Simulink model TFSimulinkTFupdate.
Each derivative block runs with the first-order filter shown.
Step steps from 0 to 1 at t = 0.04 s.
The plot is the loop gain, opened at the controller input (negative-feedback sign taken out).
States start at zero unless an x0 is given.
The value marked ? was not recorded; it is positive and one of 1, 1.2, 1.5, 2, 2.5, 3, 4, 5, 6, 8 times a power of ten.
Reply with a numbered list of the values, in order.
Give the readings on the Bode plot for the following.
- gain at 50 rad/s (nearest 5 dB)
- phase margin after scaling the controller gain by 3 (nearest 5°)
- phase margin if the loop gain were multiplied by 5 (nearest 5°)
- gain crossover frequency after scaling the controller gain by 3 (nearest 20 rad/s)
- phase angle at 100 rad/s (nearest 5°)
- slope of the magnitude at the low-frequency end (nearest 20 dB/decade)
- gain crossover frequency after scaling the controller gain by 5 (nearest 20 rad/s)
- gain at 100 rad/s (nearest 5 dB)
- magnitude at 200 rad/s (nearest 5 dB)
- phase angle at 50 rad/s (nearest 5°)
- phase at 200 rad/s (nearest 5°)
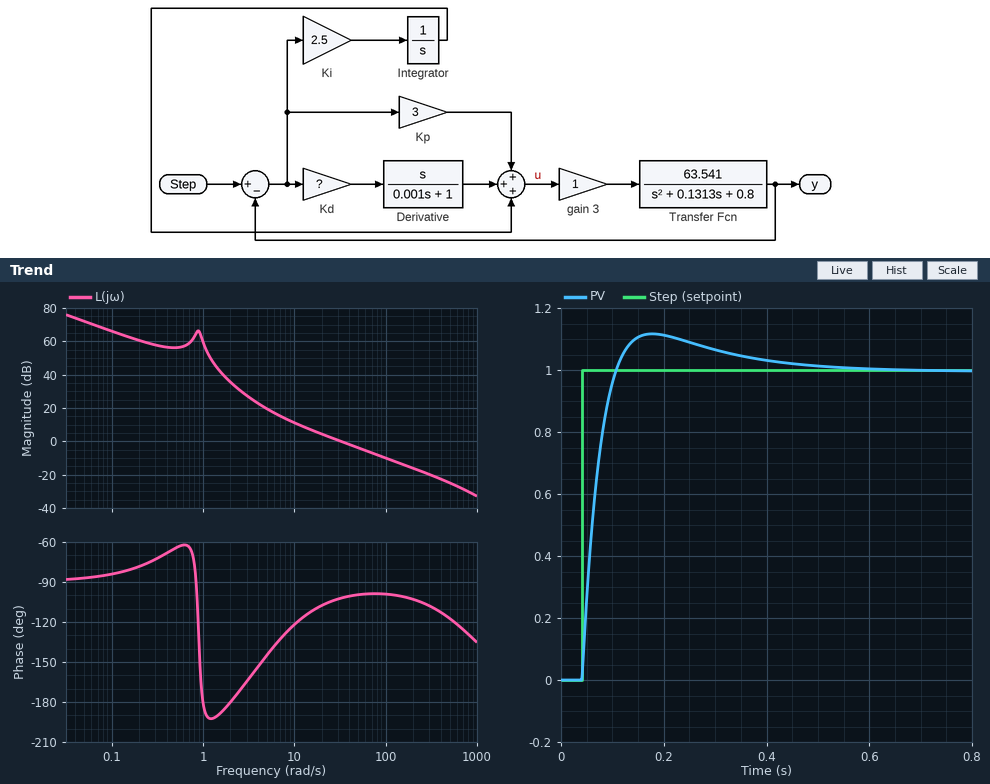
1. -5 dB
2. 80°
3. 80°
4. 100 rad/s
5. -100°
6. -20 dB/decade
7. 160 rad/s
8. -10 dB
9. -15 dB
10. -100°
11. -105°
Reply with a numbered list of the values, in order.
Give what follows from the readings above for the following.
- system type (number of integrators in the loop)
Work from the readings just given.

1. 1
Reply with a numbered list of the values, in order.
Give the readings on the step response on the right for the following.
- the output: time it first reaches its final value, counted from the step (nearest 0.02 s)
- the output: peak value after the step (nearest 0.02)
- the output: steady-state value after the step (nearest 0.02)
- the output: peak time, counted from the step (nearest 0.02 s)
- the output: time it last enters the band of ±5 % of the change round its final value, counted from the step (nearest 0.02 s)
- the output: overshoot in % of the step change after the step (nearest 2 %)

1. 0.06 s
2. 1.12
3. 1.00
4. 0.14 s
5. 0.30 s
6. 12 %
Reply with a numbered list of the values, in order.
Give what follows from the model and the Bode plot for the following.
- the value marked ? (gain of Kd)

1. 0.5
